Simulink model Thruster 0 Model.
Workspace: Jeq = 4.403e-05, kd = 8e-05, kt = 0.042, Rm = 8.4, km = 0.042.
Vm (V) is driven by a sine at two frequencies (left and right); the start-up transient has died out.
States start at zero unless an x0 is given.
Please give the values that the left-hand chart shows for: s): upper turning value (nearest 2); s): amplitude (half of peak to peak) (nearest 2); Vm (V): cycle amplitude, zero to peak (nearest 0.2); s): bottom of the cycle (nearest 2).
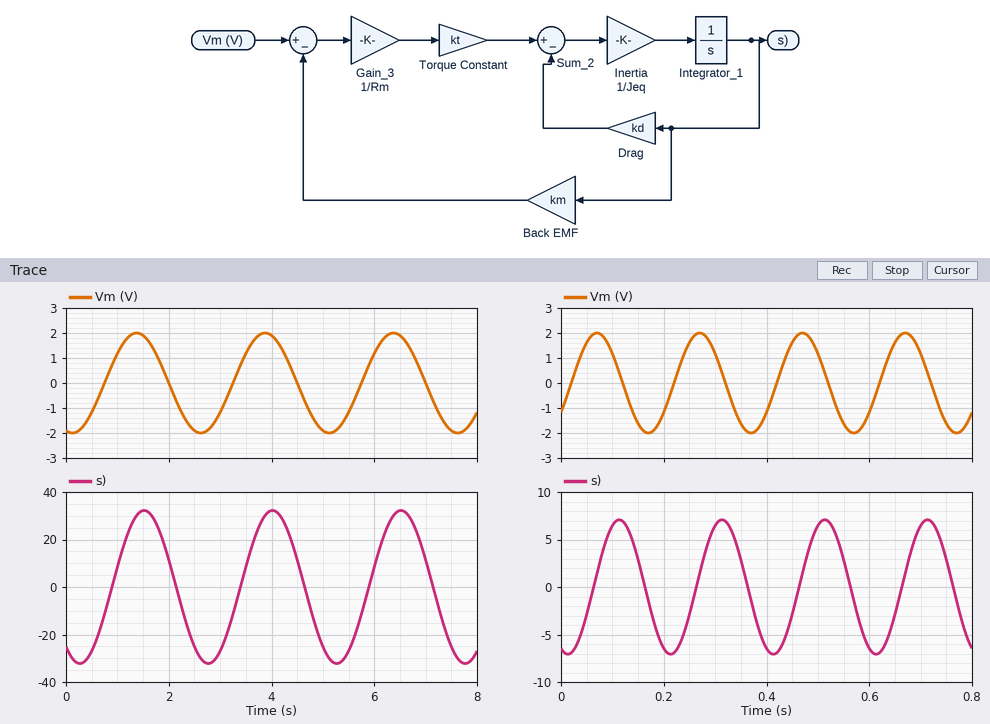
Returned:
32
32
2.0
-32
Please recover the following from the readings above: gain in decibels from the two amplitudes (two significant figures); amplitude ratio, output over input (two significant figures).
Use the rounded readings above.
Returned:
24 dB
16
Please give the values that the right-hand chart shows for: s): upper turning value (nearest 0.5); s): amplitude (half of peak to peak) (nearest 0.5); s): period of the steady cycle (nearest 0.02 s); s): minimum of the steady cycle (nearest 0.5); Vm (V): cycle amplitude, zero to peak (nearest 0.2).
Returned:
7.0
7.0
0.20 s
-7.0
2.0
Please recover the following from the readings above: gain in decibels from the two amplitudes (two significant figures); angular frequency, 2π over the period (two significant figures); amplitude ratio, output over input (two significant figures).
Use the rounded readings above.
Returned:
11 dB
31 rad/s
3.5
